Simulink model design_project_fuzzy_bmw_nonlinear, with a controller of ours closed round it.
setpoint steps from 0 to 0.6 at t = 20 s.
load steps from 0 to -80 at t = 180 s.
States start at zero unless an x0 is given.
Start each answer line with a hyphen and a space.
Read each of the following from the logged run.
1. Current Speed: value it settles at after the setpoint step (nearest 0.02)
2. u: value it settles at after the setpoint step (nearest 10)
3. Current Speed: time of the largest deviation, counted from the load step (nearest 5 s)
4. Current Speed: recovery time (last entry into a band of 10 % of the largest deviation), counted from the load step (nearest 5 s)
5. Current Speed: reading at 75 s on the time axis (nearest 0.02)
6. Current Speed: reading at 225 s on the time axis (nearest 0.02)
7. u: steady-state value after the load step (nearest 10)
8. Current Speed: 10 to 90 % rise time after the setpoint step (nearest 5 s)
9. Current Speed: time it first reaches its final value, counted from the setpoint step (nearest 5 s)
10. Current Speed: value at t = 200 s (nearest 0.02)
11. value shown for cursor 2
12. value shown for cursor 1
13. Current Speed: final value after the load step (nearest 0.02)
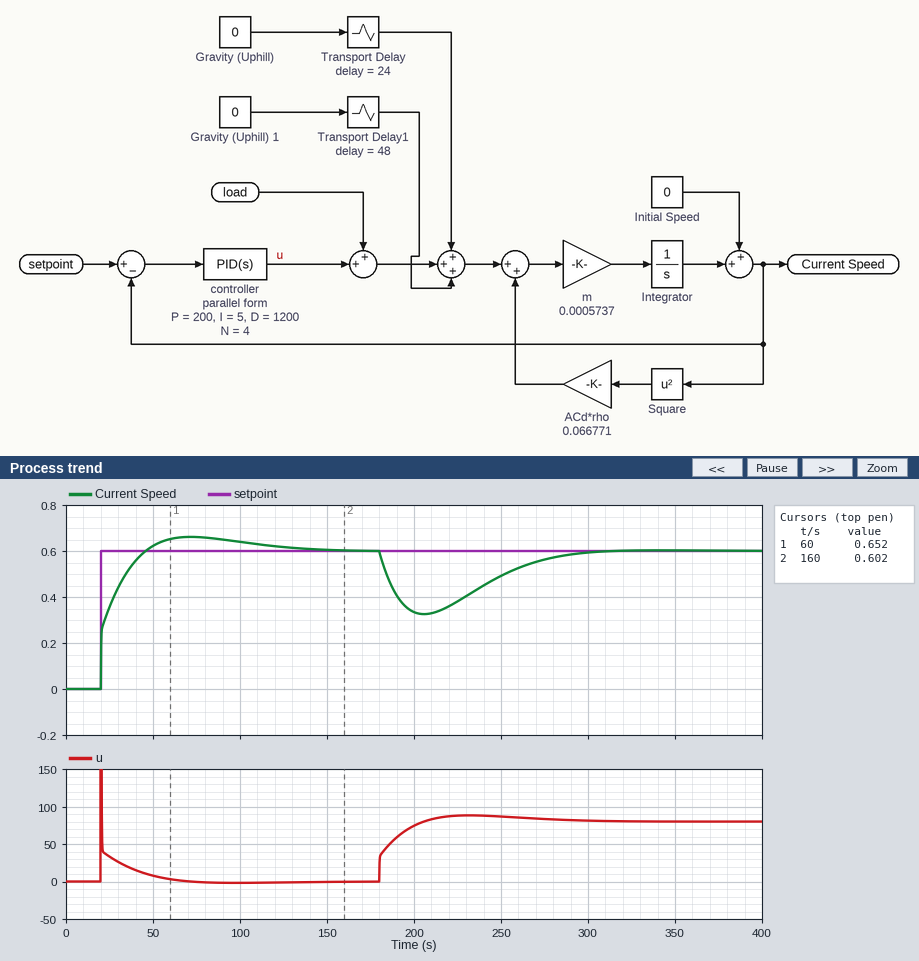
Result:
- 0.60
- 0
- 25 s
- 100 s
- 0.66
- 0.38
- 80
- 20 s
- 25 s
- 0.34
- 0.602
- 0.652
- 0.60
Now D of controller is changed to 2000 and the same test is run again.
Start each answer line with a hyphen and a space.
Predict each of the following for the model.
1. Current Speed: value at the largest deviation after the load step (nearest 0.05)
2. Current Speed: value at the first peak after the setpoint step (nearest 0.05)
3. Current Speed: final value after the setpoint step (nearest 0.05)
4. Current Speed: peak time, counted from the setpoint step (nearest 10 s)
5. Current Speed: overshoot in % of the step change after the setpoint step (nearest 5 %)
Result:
- 0.35
- 0.65
- 0.60
- 60 s
- 10 %
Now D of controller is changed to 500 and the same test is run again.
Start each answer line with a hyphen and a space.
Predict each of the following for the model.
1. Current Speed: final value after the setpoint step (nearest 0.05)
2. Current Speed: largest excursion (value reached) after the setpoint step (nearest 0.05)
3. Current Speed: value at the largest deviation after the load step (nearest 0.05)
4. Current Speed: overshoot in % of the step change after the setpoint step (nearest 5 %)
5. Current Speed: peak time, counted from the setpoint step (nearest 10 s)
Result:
- 0.60
- 0.65
- 0.30
- 10 %
- 40 s
